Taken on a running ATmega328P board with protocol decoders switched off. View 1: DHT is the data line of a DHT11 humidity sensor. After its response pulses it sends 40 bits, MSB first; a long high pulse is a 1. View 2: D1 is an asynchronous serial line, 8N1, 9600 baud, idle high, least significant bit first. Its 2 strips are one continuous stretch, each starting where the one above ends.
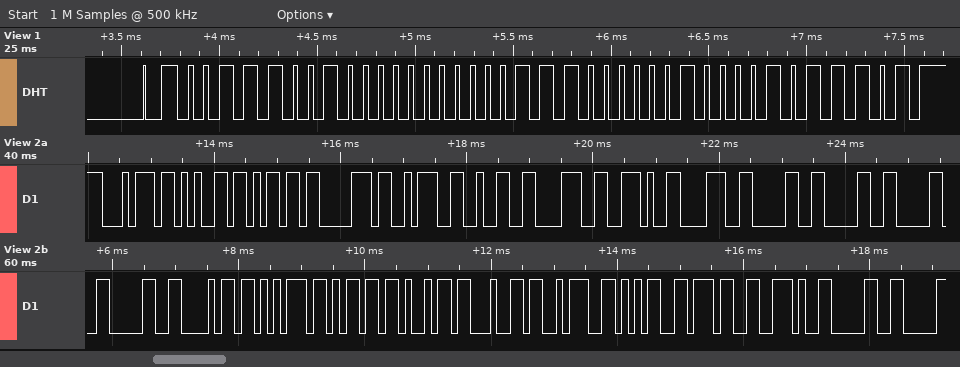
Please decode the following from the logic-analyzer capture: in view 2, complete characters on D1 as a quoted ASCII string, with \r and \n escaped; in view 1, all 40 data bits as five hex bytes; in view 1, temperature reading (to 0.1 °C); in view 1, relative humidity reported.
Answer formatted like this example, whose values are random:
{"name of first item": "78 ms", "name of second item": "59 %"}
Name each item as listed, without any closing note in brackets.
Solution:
{"in view 2, complete characters on D1 as a quoted ASCII string, with \\r and \\n escaped": "\"temp:28.80000humid:57.0\"", "in view 1, all 40 data bits as five hex bytes": "39 00 1C 08 5D", "in view 1, temperature reading": "28.8 °C", "in view 1, relative humidity reported": "57 %"}
